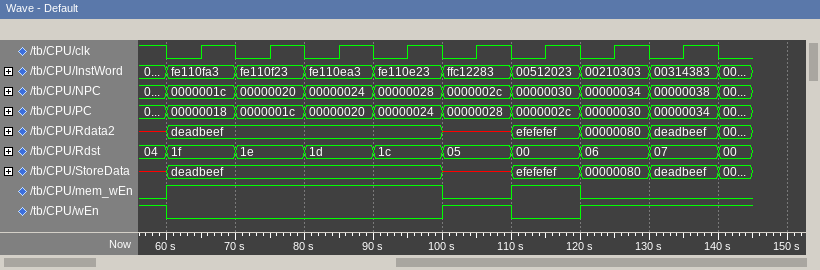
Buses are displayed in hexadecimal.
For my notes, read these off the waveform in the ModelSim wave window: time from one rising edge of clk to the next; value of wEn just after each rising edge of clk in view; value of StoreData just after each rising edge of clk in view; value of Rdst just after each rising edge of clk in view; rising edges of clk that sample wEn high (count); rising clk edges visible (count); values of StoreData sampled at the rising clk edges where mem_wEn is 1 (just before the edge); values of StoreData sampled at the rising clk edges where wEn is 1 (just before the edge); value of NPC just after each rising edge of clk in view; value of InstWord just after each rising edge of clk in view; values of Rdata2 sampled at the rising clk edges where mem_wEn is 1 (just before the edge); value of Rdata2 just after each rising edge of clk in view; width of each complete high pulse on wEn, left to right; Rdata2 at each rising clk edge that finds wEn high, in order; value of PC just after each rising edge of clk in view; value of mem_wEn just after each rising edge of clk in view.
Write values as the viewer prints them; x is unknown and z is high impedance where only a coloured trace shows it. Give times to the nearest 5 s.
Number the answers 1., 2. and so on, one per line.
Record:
1. 10 s
2. 0 0 0 0 1 0 1 1
3. deadbeef, deadbeef, deadbeef, deadbeef, x, efefefef, 00000080, deadbeef
4. 1f, 1e, 1d, 1c, 05, 00, 06, 07
5. 3
6. 8
7. deadbeef, deadbeef, deadbeef, deadbeef, efefefef
8. x, 00000080, deadbeef
9. 0000001c, 00000020, 00000024, 00000028, 0000002c, 00000030, 00000034, 00000038
10. fe110fa3, fe110f23, fe110ea3, fe110e23, ffc12283, 00512023, 00210303, 00314383
11. deadbeef, deadbeef, deadbeef, deadbeef, efefefef
12. deadbeef, deadbeef, deadbeef, deadbeef, x, efefefef, 00000080, deadbeef
13. 10 s
14. x, 00000080, deadbeef
15. 00000018, 0000001c, 00000020, 00000024, 00000028, 0000002c, 00000030, 00000034
16. 1 1 1 1 0 1 0 0
